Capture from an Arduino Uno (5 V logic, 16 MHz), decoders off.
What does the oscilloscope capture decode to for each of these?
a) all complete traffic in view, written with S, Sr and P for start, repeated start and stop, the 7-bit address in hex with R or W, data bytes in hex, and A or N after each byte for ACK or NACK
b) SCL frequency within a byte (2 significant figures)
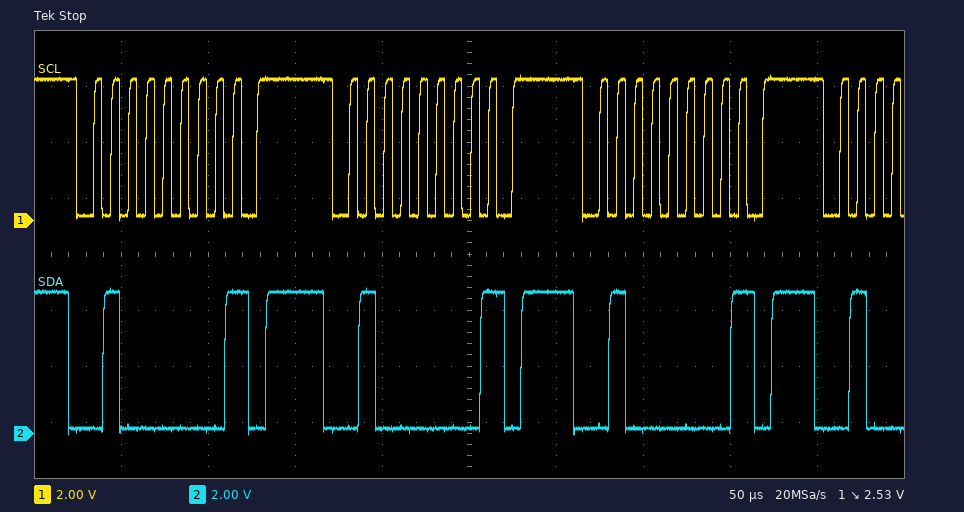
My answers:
S 20W N P S 20W N P S 20W N P
100 kHz
